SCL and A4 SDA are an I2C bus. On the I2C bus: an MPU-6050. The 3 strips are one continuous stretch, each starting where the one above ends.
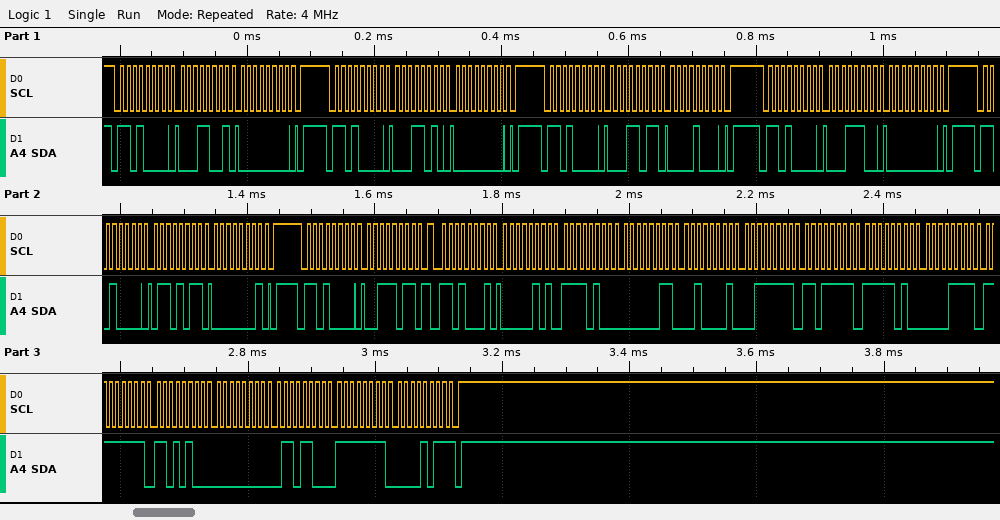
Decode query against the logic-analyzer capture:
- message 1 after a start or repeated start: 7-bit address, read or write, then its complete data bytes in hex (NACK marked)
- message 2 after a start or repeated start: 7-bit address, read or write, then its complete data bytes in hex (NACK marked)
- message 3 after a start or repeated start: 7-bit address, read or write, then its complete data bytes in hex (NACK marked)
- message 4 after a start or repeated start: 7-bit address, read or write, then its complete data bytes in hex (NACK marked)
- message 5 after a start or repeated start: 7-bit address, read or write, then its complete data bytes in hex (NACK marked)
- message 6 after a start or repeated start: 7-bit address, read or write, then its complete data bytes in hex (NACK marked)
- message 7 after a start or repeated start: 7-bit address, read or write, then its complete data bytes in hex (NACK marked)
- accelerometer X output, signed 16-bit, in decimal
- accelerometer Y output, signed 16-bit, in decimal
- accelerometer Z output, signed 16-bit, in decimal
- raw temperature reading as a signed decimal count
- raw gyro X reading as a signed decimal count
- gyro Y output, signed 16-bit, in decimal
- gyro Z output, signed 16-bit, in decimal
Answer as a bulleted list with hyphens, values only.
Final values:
- 0x68 write: 19 00
- 0x68 write: 1A 00
- 0x68 write: 1B 08
- 0x68 write: 1C 00
- 0x68 write: 6B 01
- 0x68 write: 3B
- 0x68 read: 05 F4 03 21 3F DF FA 0F FF D4 00 6C FF 0B NACK
- 1524
- 801
- 16351
- -1521
- -44
- 108
- -245
